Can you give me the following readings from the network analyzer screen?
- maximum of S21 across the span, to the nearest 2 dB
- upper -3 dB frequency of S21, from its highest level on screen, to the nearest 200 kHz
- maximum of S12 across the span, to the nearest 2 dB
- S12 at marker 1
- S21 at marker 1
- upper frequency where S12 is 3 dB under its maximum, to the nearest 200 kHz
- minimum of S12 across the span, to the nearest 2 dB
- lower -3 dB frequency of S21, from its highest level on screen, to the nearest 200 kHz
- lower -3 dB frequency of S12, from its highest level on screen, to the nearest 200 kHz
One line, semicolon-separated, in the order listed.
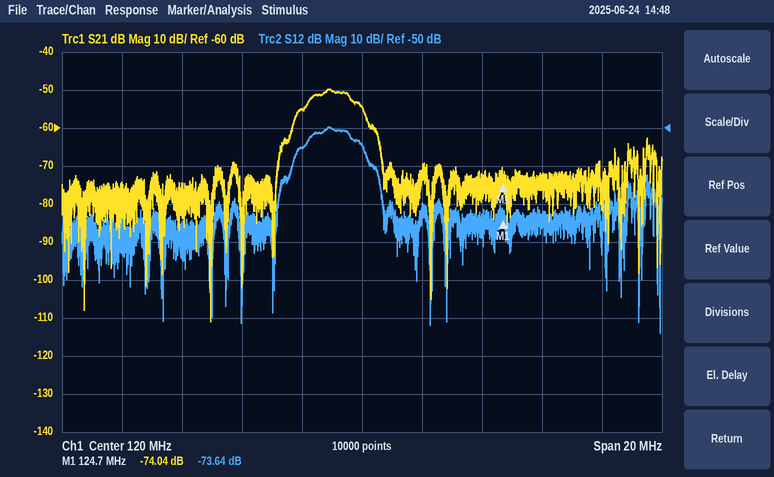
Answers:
-50 dB; 119.6 MHz; -50 dB; -73.64 dB; -74.04 dB; 119.6 MHz; -104 dB; 118.2 MHz; 118.2 MHz
